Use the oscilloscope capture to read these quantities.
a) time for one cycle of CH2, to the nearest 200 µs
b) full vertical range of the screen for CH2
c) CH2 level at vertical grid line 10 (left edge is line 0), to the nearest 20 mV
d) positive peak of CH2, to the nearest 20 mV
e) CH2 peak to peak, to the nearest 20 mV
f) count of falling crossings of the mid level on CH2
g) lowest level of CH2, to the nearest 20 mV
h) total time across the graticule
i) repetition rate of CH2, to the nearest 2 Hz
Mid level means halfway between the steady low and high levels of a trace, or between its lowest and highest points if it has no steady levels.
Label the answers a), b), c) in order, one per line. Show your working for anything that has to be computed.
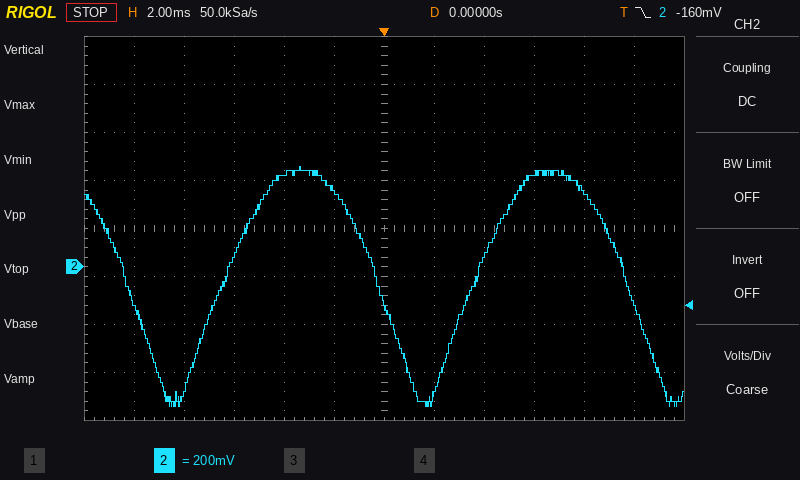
a) 10.0 ms
b) 1.6 V
c) 320 mV
d) 420 mV
e) 420 mV − (-580 mV) = 1.00 V
f) 3
g) -580 mV
h) 24 ms
i) 1 / 10.0 ms ≈ 100 Hz
